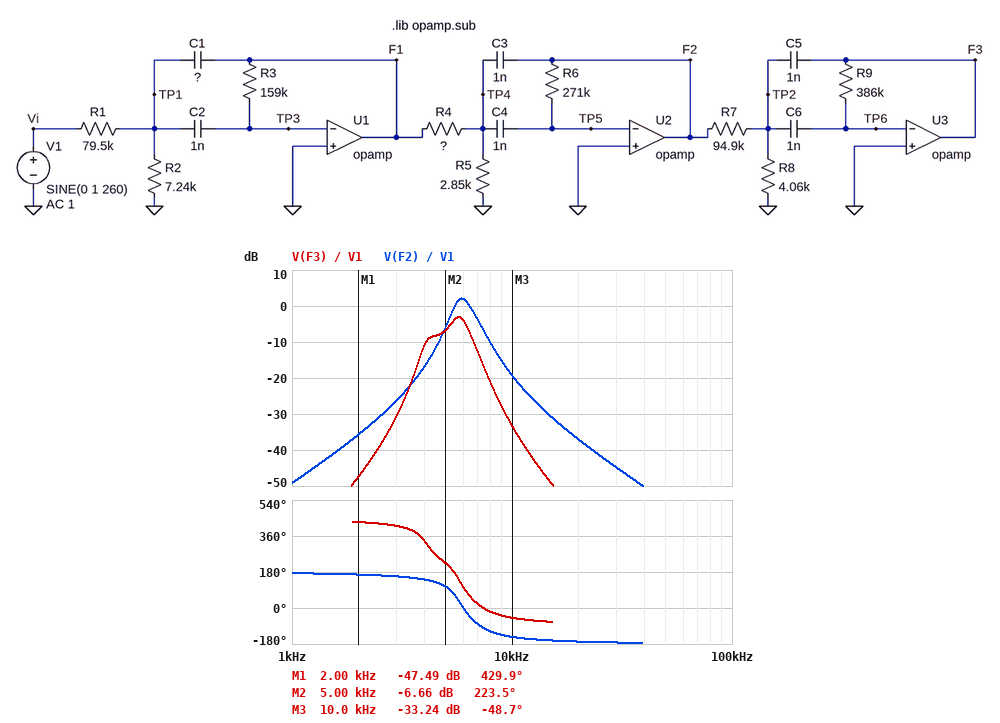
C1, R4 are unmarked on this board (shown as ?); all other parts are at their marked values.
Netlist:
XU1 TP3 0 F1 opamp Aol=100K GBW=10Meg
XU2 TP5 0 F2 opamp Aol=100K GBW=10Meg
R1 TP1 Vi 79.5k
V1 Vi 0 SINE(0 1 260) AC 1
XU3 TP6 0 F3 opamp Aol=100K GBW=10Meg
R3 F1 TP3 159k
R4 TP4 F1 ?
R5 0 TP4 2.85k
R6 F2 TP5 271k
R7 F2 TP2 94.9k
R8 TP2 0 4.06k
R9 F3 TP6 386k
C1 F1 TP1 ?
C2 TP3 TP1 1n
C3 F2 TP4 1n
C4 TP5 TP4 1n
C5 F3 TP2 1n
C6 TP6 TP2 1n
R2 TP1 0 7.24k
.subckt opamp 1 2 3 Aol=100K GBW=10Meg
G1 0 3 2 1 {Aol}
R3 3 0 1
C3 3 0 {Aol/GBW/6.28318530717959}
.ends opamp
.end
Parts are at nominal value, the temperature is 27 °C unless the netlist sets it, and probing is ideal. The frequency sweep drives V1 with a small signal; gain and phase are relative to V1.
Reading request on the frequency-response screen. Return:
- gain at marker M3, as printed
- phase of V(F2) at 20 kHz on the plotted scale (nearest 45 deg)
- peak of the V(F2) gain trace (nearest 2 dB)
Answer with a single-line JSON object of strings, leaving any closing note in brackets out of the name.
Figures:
{"gain at marker M3, as printed": "-33.24 dB", "phase of V(F2) at 20 kHz on the plotted scale": "-180 deg", "peak of the V(F2) gain trace": "2 dB"}
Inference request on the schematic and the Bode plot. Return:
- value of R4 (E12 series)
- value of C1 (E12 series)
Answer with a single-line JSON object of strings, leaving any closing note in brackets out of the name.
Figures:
{"value of R4": "120 kΩ", "value of C1": "560 pF"}
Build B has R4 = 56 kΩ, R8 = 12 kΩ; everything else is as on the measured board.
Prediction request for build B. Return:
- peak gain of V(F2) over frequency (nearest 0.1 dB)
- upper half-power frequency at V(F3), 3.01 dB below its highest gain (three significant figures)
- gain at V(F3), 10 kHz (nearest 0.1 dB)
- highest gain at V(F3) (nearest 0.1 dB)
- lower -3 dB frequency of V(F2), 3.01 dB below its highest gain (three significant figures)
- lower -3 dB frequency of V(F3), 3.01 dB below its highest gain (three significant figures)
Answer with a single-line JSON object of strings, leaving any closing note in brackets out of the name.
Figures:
{"peak gain of V(F2) over frequency": "8.9 dB", "upper half-power frequency at V(F3), 3.01 dB below its highest gain": "6.45 kHz", "gain at V(F3), 10 kHz": "-27.5 dB", "highest gain at V(F3)": "-0.5 dB", "lower -3 dB frequency of V(F2), 3.01 dB below its highest gain": "5.48 kHz", "lower -3 dB frequency of V(F3), 3.01 dB below its highest gain": "5.37 kHz"}
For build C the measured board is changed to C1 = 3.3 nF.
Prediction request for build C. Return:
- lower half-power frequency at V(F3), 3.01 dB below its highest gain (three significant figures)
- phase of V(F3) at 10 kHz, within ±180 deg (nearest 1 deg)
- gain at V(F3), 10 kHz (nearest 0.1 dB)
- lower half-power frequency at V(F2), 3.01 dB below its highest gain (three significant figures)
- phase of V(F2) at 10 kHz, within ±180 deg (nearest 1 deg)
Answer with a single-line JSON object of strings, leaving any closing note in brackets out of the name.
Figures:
{"lower half-power frequency at V(F3), 3.01 dB below its highest gain": "3.75 kHz", "phase of V(F3) at 10 kHz, within ±180 deg": "-67 deg", "gain at V(F3), 10 kHz": "-52.0 dB", "lower half-power frequency at V(F2), 3.01 dB below its highest gain": "5.01 kHz", "phase of V(F2) at 10 kHz, within ±180 deg": "-162 deg"}
